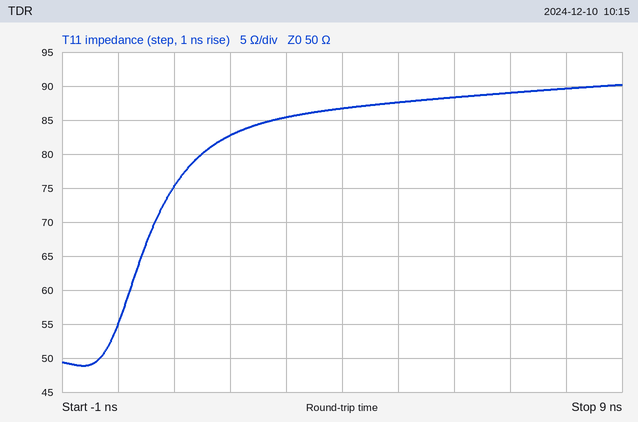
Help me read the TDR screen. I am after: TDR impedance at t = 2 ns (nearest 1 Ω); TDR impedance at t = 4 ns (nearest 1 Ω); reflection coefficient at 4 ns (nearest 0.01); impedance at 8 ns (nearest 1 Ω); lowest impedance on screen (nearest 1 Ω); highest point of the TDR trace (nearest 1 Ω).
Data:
83 Ω
87 Ω
+0.27
90 Ω
49 Ω
90 Ω
